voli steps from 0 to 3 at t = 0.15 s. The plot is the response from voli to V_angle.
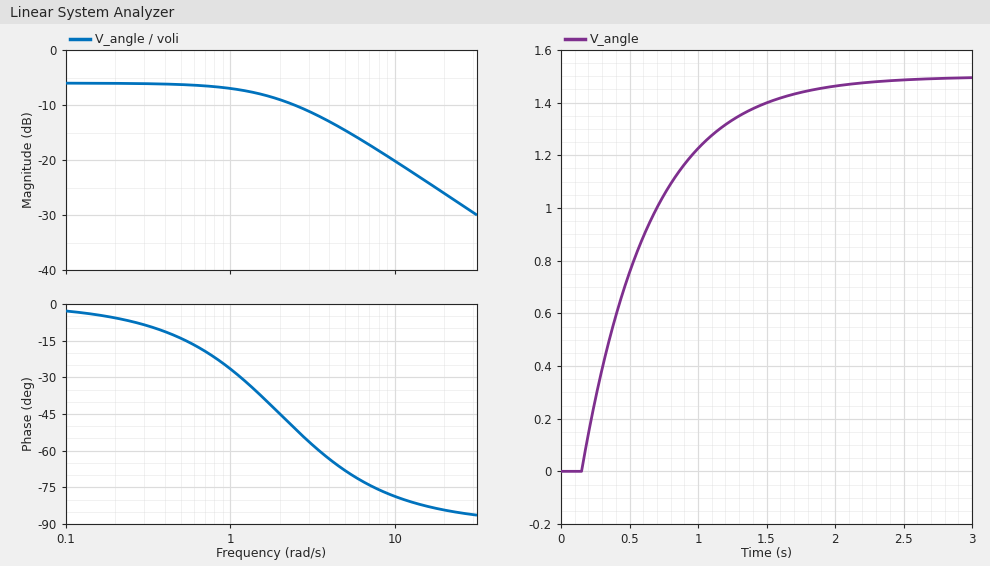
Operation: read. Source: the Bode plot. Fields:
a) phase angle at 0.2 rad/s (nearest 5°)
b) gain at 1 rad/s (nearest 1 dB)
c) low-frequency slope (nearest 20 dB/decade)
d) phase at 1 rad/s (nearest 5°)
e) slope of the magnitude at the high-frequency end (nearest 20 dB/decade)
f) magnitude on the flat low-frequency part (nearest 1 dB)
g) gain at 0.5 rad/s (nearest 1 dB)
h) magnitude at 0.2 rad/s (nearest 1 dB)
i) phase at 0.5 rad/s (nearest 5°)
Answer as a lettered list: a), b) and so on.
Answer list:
a) -5°
b) -7 dB
c) 0 dB/decade
d) -25°
e) -20 dB/decade
f) -6 dB
g) -6 dB
h) -6 dB
i) -15°
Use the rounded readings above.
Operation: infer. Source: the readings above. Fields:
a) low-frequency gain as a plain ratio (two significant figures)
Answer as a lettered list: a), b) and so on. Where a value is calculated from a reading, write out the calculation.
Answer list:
a) 10^(-6 / 20) = 0.50
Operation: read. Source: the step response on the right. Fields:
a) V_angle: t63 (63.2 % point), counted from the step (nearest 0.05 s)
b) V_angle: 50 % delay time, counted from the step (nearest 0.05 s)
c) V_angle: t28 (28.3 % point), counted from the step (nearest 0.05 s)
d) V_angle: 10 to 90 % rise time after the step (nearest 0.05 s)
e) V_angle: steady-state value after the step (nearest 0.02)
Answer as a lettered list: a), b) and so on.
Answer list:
a) 0.50 s
b) 0.35 s
c) 0.15 s
d) 1.10 s
e) 1.50
